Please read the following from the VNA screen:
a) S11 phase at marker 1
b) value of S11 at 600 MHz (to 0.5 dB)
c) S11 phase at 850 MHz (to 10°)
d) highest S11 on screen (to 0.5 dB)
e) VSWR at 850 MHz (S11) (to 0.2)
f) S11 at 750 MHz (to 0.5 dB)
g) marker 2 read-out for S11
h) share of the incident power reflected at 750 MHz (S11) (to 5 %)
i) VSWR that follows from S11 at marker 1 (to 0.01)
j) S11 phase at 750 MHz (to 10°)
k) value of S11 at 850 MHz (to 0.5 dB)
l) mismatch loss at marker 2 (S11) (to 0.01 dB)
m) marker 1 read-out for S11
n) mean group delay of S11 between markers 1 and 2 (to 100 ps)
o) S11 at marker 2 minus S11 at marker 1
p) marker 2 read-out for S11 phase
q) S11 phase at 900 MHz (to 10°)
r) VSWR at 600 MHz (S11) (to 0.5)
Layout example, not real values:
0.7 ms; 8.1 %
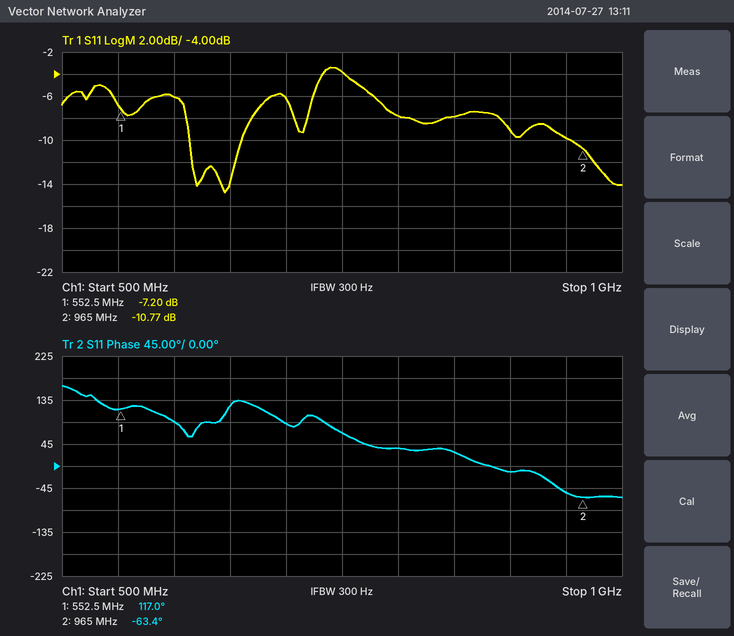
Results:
117.0°; -6.0 dB; 30°; -3.5 dB; 2.4; -4.0 dB; -10.77 dB; 40 %; 2.55; 70°; -8.0 dB; 0.38 dB; -7.20 dB; 1.2 ns; -3.57 dB; -63.4°; -10°; 3.0
